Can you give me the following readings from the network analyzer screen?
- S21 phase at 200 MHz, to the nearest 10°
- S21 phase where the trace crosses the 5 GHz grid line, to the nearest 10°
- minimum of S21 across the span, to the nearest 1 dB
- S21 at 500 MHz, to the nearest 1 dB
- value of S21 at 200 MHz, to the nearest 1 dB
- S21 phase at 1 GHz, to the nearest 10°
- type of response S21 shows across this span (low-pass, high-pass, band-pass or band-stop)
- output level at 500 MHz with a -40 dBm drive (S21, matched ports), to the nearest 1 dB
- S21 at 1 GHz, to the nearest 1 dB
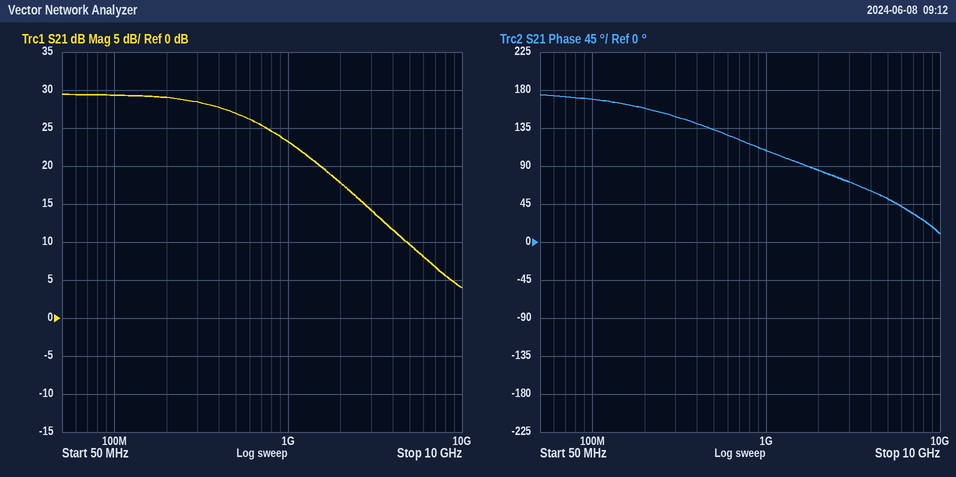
160°
50°
4 dB
27 dB
29 dB
110°
low-pass
-13 dBm
23 dB
